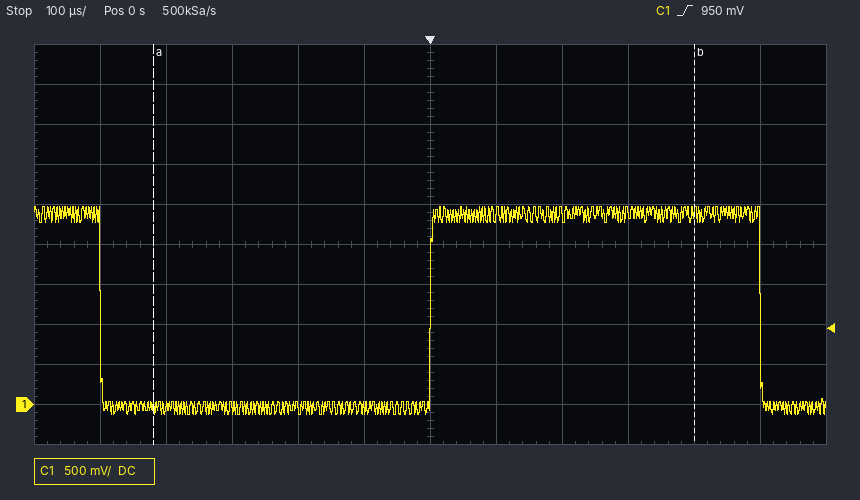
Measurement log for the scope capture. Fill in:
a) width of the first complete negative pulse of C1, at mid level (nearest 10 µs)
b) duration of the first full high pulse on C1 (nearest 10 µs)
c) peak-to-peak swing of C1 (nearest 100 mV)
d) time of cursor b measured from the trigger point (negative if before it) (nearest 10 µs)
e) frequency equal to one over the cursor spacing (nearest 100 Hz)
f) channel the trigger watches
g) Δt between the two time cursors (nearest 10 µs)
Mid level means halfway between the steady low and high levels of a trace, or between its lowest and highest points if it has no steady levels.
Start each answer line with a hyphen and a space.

- 500 µs
- 500 µs
- 2.60 V
- +400 µs
- 1.2 kHz
- C1
- 820 µs
